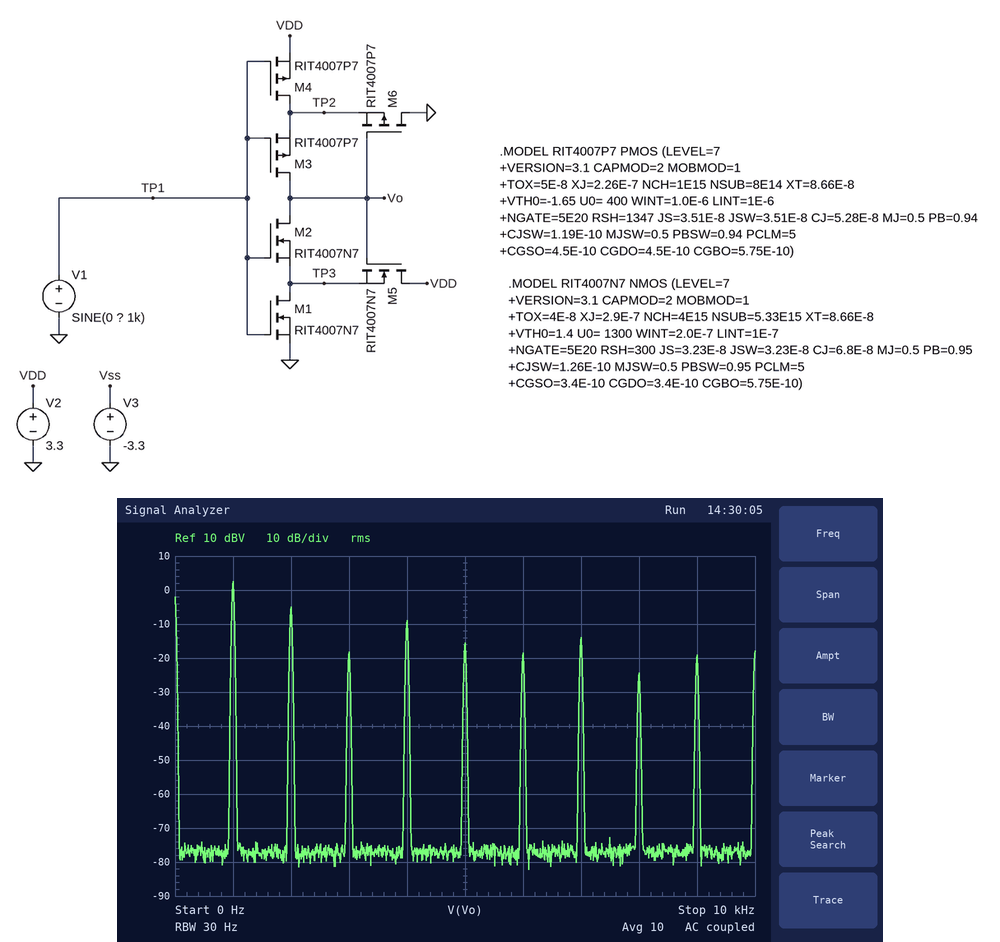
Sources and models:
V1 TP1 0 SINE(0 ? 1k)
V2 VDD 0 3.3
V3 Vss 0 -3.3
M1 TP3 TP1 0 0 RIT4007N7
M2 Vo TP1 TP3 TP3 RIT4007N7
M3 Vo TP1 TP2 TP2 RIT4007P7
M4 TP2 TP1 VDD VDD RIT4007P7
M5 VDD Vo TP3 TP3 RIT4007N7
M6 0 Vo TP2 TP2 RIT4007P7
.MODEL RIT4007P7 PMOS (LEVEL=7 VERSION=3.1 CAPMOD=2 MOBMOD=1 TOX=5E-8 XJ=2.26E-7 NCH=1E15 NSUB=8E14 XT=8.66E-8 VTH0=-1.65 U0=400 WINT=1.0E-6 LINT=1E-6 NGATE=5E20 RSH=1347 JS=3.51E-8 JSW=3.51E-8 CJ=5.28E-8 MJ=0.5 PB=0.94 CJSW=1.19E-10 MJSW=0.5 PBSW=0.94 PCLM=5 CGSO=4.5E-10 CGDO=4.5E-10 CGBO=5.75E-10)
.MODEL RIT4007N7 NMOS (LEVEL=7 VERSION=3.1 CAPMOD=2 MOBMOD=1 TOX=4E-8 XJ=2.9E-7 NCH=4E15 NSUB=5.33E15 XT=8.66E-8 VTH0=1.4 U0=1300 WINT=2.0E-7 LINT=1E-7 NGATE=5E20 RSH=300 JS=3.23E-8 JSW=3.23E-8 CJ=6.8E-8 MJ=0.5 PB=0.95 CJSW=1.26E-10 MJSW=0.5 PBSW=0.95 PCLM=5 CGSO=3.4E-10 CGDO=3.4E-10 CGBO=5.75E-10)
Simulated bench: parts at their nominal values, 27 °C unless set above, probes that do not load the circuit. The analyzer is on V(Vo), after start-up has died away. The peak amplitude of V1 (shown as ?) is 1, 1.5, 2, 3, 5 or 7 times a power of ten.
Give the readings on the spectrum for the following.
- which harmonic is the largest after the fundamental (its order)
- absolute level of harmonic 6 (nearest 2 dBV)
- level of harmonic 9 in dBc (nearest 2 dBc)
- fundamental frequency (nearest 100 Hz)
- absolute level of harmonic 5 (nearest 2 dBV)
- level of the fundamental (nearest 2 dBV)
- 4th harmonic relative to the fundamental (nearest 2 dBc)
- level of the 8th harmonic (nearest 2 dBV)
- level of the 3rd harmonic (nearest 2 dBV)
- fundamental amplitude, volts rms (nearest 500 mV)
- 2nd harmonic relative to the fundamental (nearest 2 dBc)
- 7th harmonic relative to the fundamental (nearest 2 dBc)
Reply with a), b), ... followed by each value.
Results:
a) 2
b) -18 dBV
c) -22 dBc
d) 1.0 kHz
e) -16 dBV
f) 2 dBV
g) -12 dBc
h) -24 dBV
i) -18 dBV
j) 1.5 V
k) -8 dBc
l) -16 dBc
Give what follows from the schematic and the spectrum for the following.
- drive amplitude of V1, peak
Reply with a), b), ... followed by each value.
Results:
a) 3 V
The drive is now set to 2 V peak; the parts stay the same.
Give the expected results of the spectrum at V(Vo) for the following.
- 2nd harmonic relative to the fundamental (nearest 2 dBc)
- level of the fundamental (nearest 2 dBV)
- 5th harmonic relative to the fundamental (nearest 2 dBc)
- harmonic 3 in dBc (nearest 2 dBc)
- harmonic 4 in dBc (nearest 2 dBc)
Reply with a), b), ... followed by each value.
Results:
a) -4 dBc
b) 2 dBV
c) -12 dBc
d) -16 dBc
e) -16 dBc
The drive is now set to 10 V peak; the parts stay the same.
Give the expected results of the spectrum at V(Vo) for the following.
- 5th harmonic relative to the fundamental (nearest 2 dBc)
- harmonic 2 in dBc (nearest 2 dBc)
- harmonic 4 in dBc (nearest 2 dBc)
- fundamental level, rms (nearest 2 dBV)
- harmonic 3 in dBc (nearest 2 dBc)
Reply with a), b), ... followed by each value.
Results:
a) -16 dBc
b) -16 dBc
c) -18 dBc
d) 4 dBV
e) -10 dBc
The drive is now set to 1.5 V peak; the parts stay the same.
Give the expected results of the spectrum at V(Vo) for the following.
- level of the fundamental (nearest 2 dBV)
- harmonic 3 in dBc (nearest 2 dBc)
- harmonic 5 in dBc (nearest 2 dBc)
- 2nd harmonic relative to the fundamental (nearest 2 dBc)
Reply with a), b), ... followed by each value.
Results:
a) -32 dBV
b) 0 dBc
c) -2 dBc
d) 0 dBc
